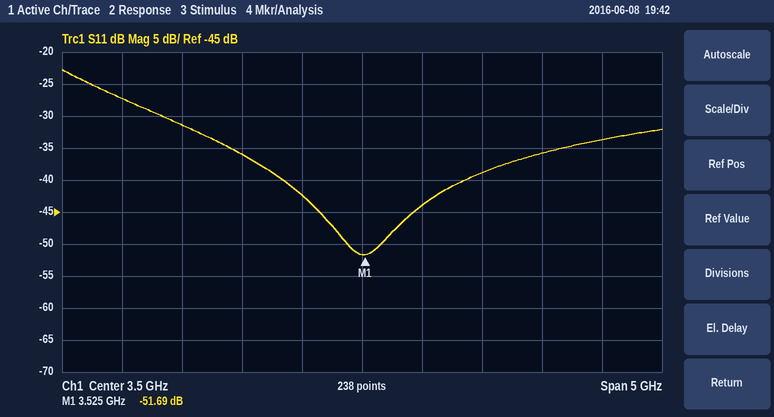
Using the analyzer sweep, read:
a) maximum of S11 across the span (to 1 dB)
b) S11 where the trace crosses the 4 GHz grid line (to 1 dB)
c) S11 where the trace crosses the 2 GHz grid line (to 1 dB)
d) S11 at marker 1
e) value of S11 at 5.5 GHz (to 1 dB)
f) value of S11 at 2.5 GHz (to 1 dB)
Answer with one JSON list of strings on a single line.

["-23 dB", "-44 dB", "-31 dB", "-51.69 dB", "-34 dB", "-36 dB"]
